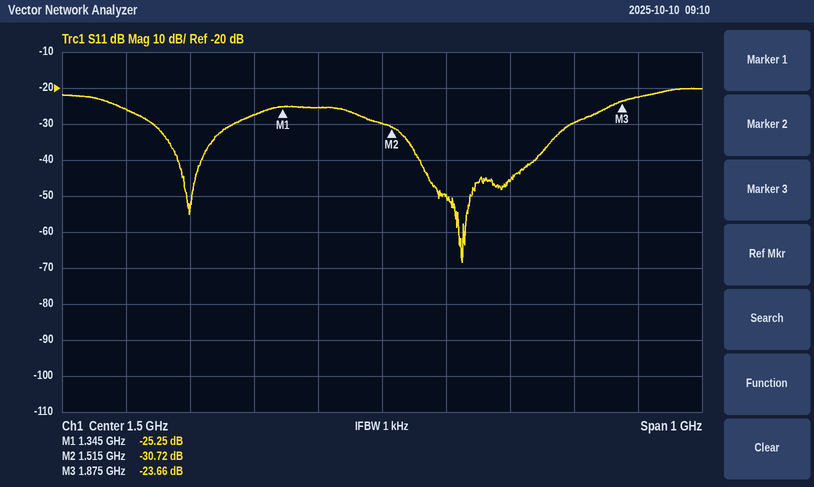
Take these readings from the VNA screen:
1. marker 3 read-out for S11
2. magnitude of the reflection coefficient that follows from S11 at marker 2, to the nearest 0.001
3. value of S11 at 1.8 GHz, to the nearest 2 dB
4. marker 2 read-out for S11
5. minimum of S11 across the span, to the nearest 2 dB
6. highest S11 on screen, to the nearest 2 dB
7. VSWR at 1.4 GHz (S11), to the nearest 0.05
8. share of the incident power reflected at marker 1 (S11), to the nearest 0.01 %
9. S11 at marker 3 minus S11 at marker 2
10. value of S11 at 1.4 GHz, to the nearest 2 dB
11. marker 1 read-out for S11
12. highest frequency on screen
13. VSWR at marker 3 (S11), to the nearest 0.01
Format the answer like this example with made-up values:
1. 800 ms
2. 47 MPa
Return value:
1. -23.66 dB
2. 0.029
3. -30 dB
4. -30.72 dB
5. -68 dB
6. -20 dB
7. 1.10
8. 0.30 %
9. 7.06 dB
10. -26 dB
11. -25.25 dB
12. 2 GHz
13. 1.14
